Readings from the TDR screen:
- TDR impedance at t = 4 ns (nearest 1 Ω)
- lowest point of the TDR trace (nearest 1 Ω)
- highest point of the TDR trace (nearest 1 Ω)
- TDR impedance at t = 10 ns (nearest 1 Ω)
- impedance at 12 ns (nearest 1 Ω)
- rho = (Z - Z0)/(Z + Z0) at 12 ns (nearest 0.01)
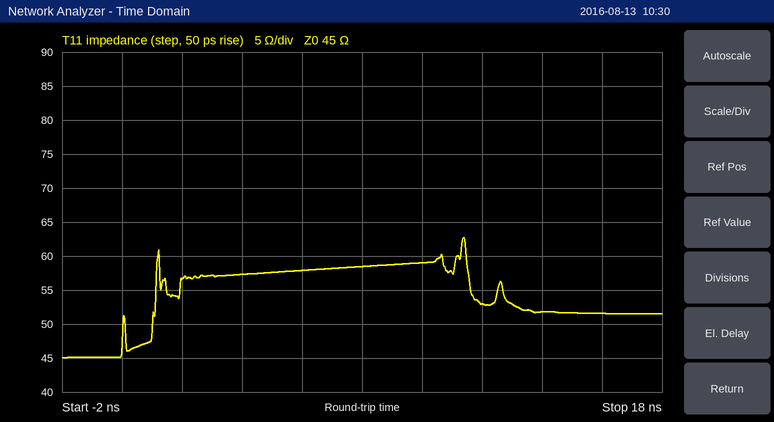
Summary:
57 Ω
45 Ω
63 Ω
59 Ω
53 Ω
+0.08
